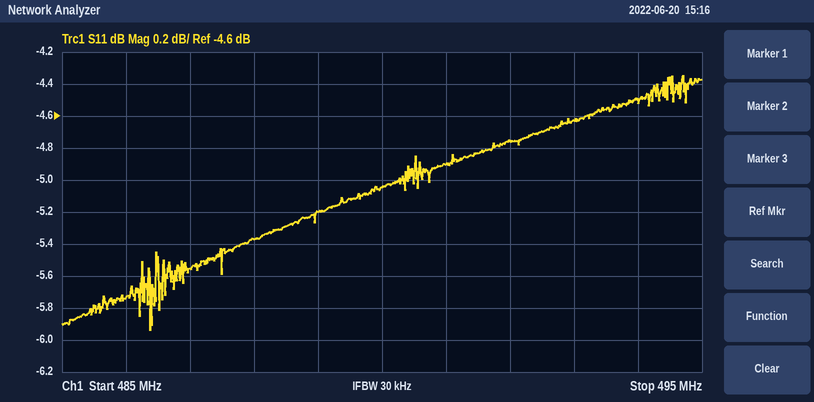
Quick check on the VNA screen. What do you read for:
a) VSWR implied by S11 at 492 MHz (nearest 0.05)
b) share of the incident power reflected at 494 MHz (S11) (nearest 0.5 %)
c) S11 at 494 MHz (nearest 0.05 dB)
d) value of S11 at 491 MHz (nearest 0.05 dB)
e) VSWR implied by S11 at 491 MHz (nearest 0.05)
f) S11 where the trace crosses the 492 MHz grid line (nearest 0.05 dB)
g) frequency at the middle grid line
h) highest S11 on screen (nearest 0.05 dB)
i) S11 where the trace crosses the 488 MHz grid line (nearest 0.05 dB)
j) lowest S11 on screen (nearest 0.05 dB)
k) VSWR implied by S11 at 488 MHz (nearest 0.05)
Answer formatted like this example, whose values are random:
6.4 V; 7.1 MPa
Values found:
3.75; 35.5 %; -4.50 dB; -4.90 dB; 3.65; -4.75 dB; 490 MHz; -4.35 dB; -5.35 dB; -5.95 dB; 3.35
